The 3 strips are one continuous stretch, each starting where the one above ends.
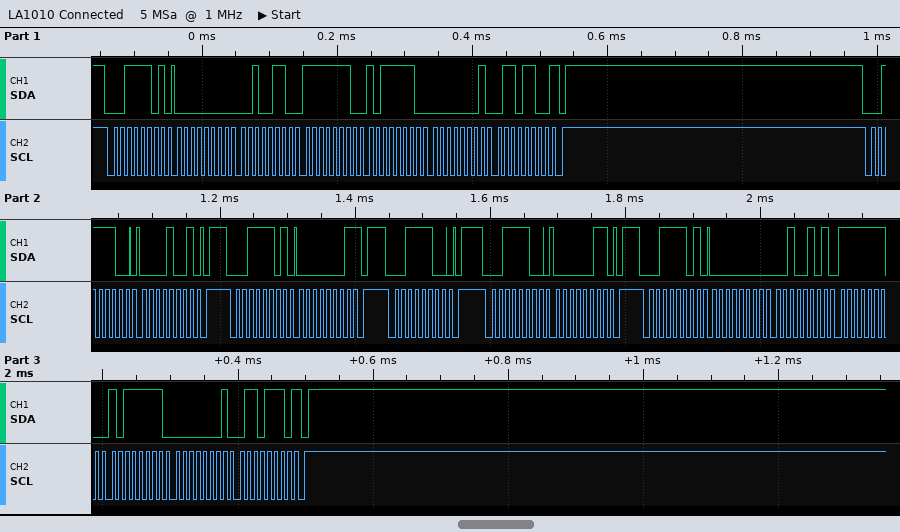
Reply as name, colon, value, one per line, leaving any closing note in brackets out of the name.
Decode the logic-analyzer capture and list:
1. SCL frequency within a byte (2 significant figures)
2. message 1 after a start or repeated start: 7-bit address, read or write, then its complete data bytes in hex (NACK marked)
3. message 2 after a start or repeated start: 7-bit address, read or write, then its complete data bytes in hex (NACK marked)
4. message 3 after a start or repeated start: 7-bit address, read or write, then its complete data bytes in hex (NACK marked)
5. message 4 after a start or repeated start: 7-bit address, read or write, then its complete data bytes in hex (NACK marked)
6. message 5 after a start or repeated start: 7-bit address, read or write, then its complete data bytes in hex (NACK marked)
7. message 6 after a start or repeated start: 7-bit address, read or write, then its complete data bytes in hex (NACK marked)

SCL frequency within a byte: 100 kHz
message 1 after a start or repeated start: 7-bit address, read or write, then its complete data bytes in hex: 0x1E read: 00 26 FE BE 01 6C NACK
message 2 after a start or repeated start: 7-bit address, read or write, then its complete data bytes in hex: 0x1E write: 09
message 3 after a start or repeated start: 7-bit address, read or write, then its complete data bytes in hex: 0x1E read: 01 NACK
message 4 after a start or repeated start: 7-bit address, read or write, then its complete data bytes in hex: 0x1E write
message 5 after a start or repeated start: 7-bit address, read or write, then its complete data bytes in hex: 0x1E write: 03
message 6 after a start or repeated start: 7-bit address, read or write, then its complete data bytes in hex: 0x1E read: 00 25 FE BF 01 6E NACK
